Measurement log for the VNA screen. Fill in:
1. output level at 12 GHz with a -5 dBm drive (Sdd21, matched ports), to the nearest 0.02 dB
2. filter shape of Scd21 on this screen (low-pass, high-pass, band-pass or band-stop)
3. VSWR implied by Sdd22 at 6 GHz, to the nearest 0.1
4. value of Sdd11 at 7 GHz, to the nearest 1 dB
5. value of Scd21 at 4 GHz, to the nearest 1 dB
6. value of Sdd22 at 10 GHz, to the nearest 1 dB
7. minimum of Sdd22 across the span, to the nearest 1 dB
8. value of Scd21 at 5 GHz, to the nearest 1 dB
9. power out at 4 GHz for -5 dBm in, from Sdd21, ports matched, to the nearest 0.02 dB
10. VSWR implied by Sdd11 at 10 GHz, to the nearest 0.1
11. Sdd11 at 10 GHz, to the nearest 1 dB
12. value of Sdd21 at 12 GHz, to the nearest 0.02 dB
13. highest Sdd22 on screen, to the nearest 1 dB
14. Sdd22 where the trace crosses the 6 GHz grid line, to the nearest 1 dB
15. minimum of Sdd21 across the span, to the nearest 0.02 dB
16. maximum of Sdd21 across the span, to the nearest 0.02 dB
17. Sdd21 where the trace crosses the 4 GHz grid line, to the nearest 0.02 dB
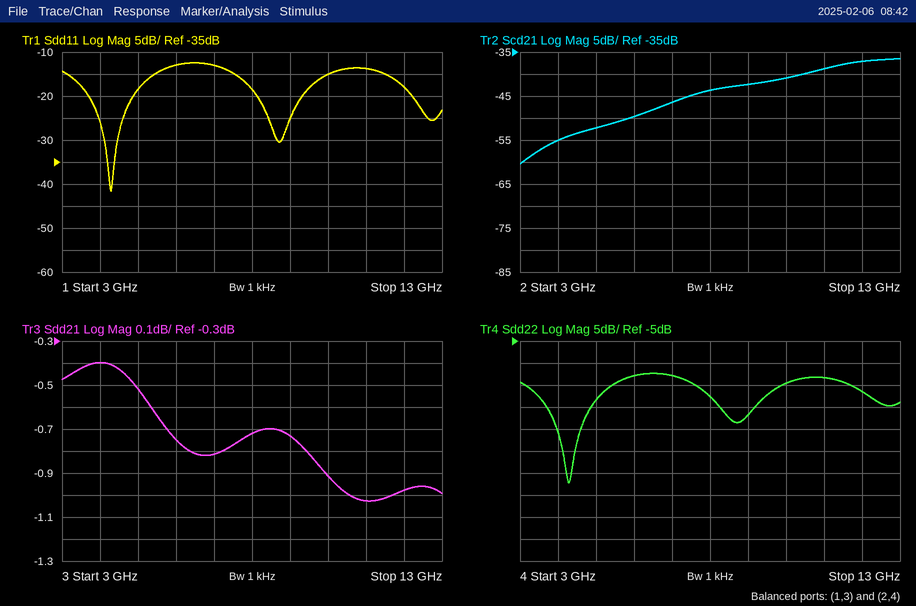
-5.98 dBm
high-pass
1.6
-13 dB
-55 dB
-15 dB
-37 dB
-52 dB
-5.40 dBm
1.4
-15 dB
-0.98 dB
-12 dB
-13 dB
-1.02 dB
-0.40 dB
-0.40 dB
